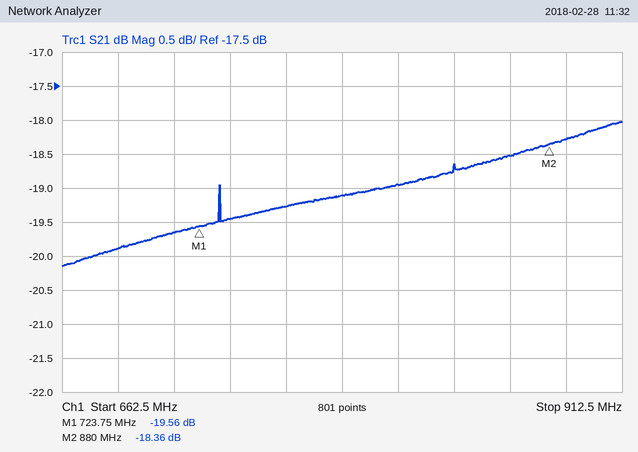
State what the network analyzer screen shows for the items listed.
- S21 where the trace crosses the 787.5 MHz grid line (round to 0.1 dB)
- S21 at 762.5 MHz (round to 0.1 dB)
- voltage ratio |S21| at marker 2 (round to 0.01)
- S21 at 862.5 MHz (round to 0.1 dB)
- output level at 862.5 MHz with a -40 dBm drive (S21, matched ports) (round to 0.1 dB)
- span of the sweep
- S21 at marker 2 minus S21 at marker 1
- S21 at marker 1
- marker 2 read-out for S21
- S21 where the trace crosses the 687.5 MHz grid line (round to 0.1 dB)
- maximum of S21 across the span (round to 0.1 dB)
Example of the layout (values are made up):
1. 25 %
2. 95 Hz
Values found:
1. -19.1 dB
2. -19.3 dB
3. 0.12
4. -18.5 dB
5. -58.5 dBm
6. 250 MHz
7. 1.20 dB
8. -19.56 dB
9. -18.36 dB
10. -19.9 dB
11. -18.0 dB
